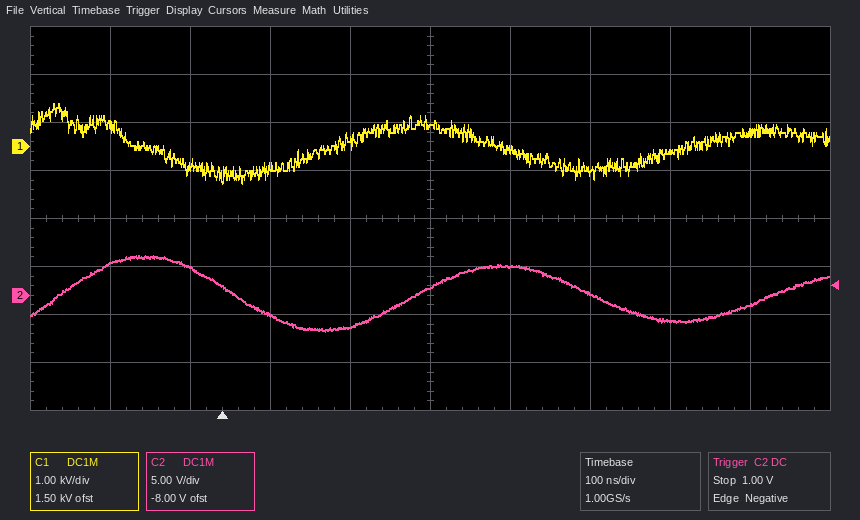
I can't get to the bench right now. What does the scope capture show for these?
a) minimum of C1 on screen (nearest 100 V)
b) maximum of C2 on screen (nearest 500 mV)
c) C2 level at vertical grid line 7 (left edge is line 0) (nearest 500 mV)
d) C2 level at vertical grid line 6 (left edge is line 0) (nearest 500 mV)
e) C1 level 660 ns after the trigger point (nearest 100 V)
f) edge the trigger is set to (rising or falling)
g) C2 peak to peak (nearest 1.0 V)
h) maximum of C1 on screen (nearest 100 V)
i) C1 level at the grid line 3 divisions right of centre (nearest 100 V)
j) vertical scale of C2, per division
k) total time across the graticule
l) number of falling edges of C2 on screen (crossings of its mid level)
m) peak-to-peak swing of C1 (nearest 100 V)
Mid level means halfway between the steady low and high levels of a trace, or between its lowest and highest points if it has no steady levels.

-800 V
4.0 V
0.0 V
3.0 V
300 V
falling
8.0 V
900 V
-100 V
5 V
1 µs
2
1.7 kV
